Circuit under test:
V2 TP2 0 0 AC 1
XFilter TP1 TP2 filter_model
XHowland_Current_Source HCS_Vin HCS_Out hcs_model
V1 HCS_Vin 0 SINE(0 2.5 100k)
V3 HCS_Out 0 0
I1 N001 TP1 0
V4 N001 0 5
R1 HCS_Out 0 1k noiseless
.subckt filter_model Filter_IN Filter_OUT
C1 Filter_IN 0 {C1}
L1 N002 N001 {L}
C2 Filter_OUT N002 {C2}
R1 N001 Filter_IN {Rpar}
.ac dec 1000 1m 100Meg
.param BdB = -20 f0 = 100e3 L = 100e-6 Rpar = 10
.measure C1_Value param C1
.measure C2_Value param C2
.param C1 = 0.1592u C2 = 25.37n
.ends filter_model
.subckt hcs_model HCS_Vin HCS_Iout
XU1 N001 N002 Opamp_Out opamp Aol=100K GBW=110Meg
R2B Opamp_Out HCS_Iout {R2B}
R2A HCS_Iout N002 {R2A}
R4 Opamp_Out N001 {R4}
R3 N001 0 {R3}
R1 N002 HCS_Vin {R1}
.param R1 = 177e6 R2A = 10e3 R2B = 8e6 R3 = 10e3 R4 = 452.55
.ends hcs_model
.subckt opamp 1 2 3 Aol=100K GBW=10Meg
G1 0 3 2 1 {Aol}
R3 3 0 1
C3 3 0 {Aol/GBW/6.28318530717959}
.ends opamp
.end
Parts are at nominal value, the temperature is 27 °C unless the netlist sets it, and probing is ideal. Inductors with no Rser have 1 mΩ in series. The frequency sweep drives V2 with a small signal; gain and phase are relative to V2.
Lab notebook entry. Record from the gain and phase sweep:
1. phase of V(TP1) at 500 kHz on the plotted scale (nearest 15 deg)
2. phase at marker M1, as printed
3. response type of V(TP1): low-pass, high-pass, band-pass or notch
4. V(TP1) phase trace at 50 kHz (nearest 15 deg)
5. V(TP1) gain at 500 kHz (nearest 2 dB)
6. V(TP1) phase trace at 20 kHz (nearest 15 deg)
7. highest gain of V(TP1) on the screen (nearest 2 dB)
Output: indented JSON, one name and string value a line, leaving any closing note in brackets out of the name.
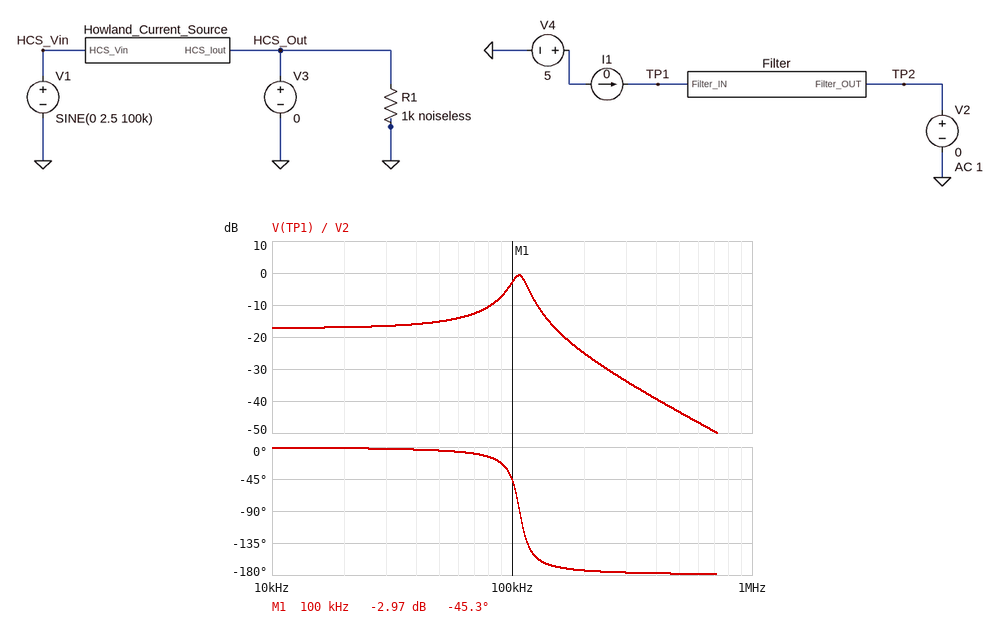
{
  "phase of V(TP1) at 500 kHz on the plotted scale": "-180 deg",
  "phase at marker M1, as printed": "-45.3 deg",
  "response type of V(TP1): low-pass, high-pass, band-pass or notch": "low-pass",
  "V(TP1) phase trace at 50 kHz": "0 deg",
  "V(TP1) gain at 500 kHz": "-44 dB",
  "V(TP1) phase trace at 20 kHz": "0 deg",
  "highest gain of V(TP1) on the screen": "0 dB"
}
